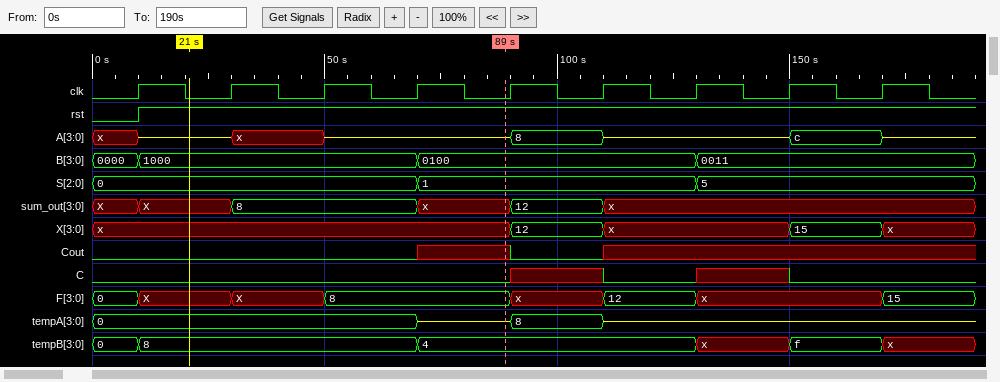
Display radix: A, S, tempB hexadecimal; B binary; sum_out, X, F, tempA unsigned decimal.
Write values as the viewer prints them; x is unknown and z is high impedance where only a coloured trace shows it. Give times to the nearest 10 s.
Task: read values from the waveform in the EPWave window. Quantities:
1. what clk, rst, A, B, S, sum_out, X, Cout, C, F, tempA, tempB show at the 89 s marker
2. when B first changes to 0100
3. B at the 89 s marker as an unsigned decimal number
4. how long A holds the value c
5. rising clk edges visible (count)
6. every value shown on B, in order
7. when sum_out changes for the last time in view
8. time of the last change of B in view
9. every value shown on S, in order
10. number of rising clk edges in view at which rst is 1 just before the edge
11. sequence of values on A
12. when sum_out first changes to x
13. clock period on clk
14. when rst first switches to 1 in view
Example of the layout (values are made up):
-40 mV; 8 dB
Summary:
clk=0, rst=1, A=z, B=0100, S=1, sum_out=x, X=x, Cout=x, C=0, F=8, tempA=z, tempB=4; 70 s; 4; 20 s; 9; 0000, 1000, 0100, 0011; 110 s; 130 s; 0, 1, 5; 8; x, z, x, z, 8, z, c, z; 70 s; 20 s; 10 s
